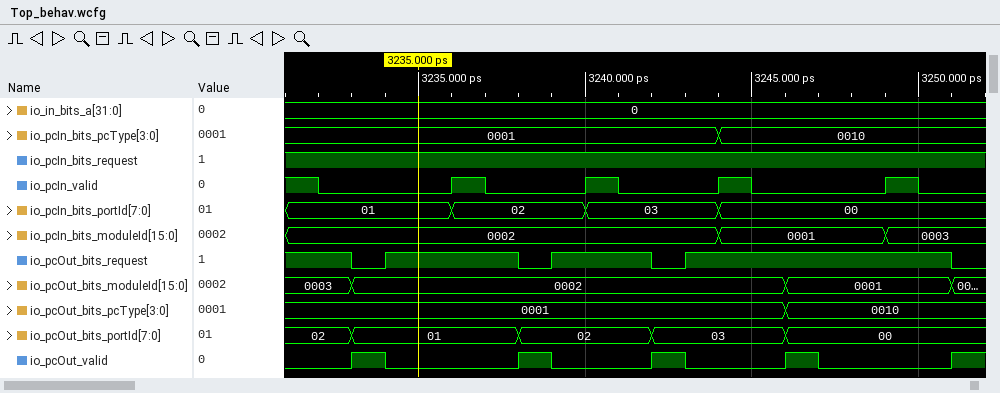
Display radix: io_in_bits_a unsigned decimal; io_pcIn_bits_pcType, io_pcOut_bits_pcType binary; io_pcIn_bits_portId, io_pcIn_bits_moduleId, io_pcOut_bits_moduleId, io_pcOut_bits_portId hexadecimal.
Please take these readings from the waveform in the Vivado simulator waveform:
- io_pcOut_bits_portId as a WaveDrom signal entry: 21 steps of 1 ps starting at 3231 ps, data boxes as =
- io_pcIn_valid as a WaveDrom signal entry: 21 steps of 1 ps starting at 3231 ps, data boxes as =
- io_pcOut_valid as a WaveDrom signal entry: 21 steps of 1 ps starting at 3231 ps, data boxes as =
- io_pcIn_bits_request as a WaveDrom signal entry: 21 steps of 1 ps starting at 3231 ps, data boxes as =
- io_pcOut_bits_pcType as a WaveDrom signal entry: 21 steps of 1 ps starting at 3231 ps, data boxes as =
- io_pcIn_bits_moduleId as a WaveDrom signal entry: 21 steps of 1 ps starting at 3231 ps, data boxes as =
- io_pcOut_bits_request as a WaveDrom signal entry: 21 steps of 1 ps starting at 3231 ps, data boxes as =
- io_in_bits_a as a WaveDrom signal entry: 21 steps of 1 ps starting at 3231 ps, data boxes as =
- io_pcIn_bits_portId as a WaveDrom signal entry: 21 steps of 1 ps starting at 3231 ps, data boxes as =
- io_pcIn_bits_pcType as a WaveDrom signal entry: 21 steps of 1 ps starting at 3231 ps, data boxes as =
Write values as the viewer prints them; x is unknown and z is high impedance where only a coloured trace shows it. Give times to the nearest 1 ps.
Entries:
{name: 'io_pcOut_bits_portId', wave: '=.=....=...=...=.....', data: '02 01 02 03 00'}
{name: 'io_pcIn_valid', wave: '10...10..10..10...10.'}
{name: 'io_pcOut_valid', wave: '0.10...10..10..10...1'}
{name: 'io_pcIn_bits_request', wave: '1....................'}
{name: 'io_pcOut_bits_pcType', wave: '=..............=.....', data: '0001 0010'}
{name: 'io_pcIn_bits_moduleId', wave: '=............=....=..', data: '0002 0001 0003'}
{name: 'io_pcOut_bits_request', wave: '1.01...01..01.......0'}
{name: 'io_in_bits_a', wave: '=....................', data: '0'}
{name: 'io_pcIn_bits_portId', wave: '=....=...=...=.......', data: '01 02 03 00'}
{name: 'io_pcIn_bits_pcType', wave: '=............=.......', data: '0001 0010'}
